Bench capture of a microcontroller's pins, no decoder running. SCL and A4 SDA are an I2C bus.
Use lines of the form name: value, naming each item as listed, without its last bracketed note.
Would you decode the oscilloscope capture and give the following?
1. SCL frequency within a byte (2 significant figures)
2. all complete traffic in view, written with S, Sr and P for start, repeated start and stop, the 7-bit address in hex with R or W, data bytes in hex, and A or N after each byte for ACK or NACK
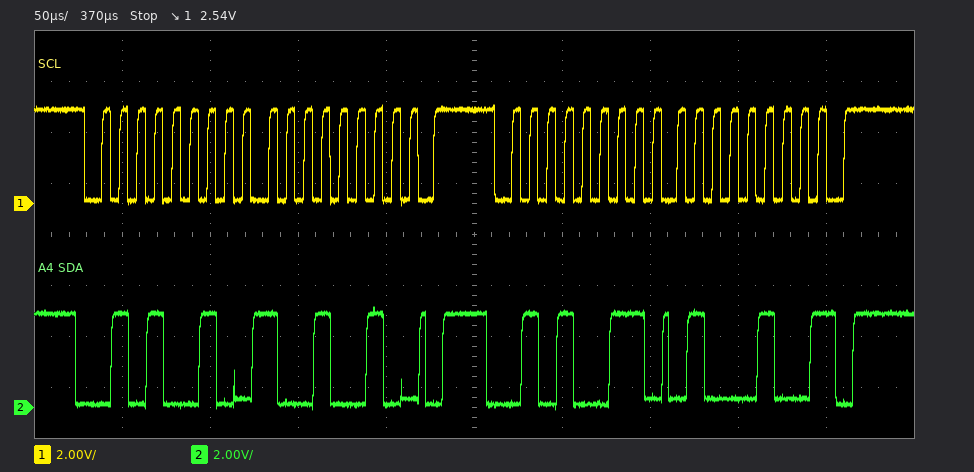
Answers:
SCL frequency within a byte: 100 kHz
all complete traffic in view, written with S, Sr and P for start, repeated start and stop, the 7-bit address in hex with R or W, data bytes in hex, and A or N after each byte for ACK or NACK: S 29W A 92 A P S 29R A 44 N P
